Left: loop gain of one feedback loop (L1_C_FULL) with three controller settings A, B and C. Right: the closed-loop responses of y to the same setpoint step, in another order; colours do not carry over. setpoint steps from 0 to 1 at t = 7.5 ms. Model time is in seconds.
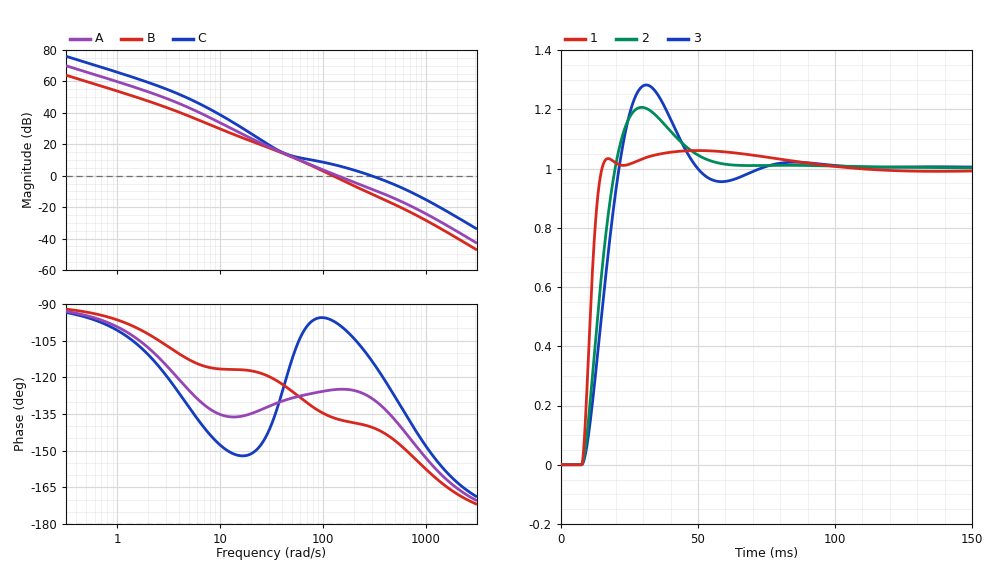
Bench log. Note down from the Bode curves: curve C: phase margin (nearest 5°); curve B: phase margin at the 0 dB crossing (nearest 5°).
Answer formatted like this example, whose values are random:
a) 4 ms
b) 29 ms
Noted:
a) 65°
b) 45°
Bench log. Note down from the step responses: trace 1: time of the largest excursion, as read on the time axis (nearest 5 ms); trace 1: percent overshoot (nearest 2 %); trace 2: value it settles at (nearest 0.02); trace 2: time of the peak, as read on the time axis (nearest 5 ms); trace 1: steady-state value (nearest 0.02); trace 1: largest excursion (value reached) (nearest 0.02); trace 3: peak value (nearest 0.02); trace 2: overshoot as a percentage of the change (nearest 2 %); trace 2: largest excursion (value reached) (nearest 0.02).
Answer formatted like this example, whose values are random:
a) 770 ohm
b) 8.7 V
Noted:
a) 50 ms
b) 6 %
c) 1.00
d) 30 ms
e) 1.00
f) 1.06
g) 1.28
h) 20 %
i) 1.20
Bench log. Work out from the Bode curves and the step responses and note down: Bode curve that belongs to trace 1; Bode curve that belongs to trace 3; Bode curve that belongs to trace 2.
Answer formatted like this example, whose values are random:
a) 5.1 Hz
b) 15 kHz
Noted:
a) C
b) B
c) A
